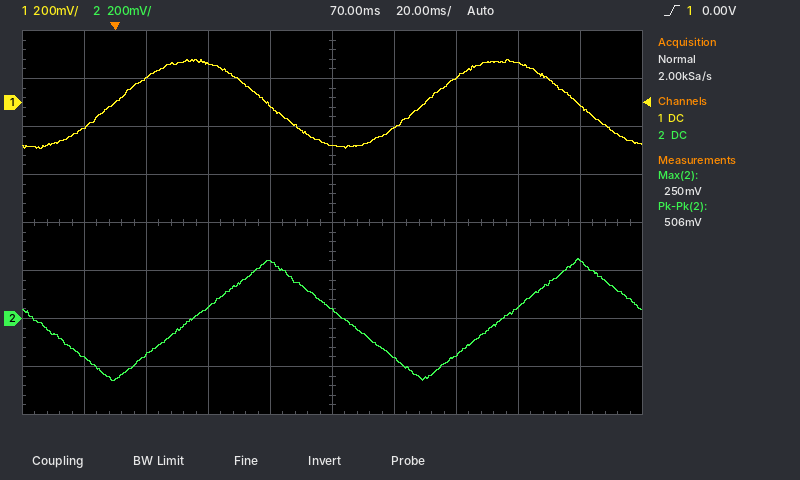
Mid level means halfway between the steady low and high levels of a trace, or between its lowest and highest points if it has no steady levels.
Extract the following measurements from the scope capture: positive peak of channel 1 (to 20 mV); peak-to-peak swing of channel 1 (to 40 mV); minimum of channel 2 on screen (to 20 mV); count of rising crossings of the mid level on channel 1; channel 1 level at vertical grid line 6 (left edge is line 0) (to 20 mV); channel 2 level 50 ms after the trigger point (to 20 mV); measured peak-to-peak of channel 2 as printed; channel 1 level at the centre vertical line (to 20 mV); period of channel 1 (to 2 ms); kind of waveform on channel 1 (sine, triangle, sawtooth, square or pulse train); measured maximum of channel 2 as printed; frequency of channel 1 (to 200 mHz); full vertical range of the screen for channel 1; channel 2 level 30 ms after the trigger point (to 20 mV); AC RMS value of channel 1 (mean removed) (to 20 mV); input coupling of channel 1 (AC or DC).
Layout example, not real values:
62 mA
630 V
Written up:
180 mV
360 mV
-260 mV
2
-100 mV
240 mV
506 mV
-180 mV
100 ms
sine
250 mV
10.0 Hz
1.6 V
40 mV
120 mV
DC
